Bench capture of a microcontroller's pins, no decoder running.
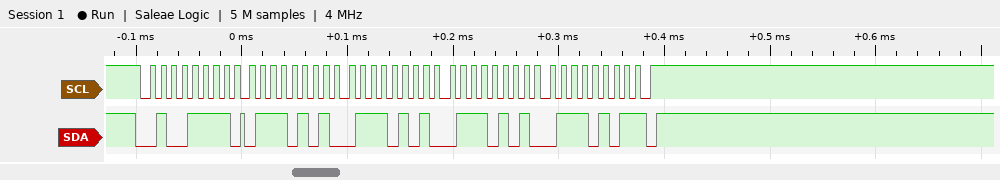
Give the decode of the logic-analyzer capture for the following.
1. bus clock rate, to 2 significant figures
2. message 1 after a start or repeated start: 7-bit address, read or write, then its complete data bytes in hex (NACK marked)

100 kHz
0x27 read: 75 75 75 75 NACK
